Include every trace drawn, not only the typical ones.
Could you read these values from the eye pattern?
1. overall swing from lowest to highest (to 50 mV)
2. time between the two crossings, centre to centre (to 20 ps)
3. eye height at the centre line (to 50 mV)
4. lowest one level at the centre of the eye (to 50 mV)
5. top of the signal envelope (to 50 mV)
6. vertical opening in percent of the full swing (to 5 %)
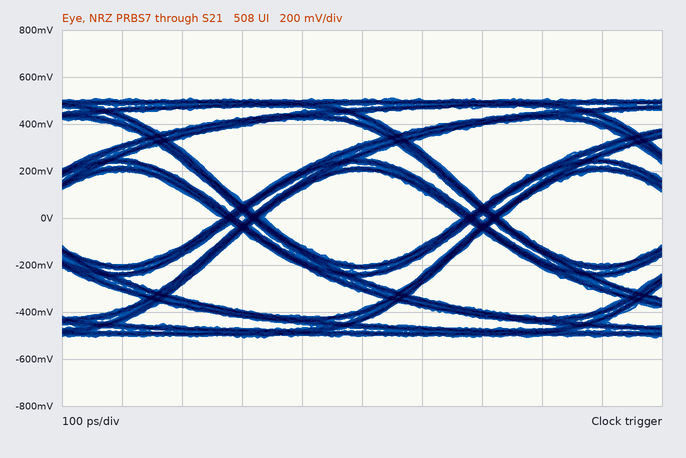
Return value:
1.00 V
400 ps
400 mV
200 mV
500 mV
40 %
